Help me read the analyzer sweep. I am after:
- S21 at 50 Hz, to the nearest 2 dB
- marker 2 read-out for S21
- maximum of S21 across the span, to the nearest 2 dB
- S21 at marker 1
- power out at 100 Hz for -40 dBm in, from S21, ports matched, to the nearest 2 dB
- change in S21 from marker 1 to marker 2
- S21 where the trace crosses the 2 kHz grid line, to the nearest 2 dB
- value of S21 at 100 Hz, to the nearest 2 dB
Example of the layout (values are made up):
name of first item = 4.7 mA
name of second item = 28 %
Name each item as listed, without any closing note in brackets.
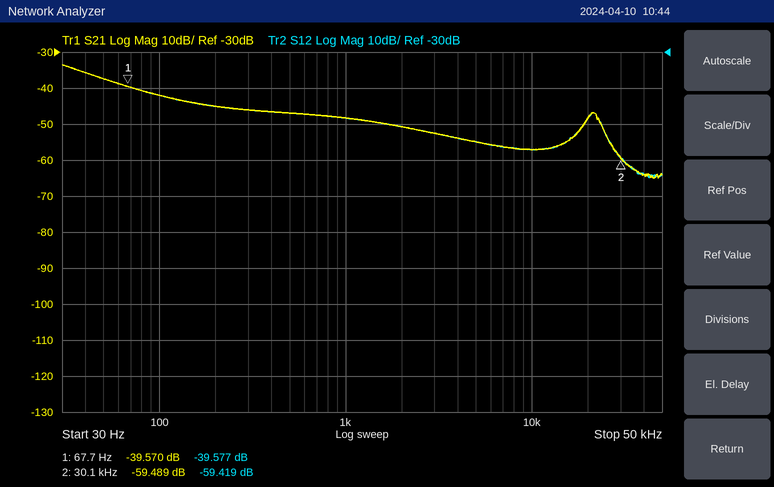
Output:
S21 at 50 Hz, to the nearest 2 dB = -38 dB
marker 2 read-out for S21 = -59.489 dB
maximum of S21 across the span, to the nearest 2 dB = -34 dB
S21 at marker 1 = -39.570 dB
power out at 100 Hz for -40 dBm in, from S21, ports matched, to the nearest 2 dB = -82 dBm
change in S21 from marker 1 to marker 2 = -19.919 dB
S21 where the trace crosses the 2 kHz grid line, to the nearest 2 dB = -50 dB
value of S21 at 100 Hz, to the nearest 2 dB = -42 dB
